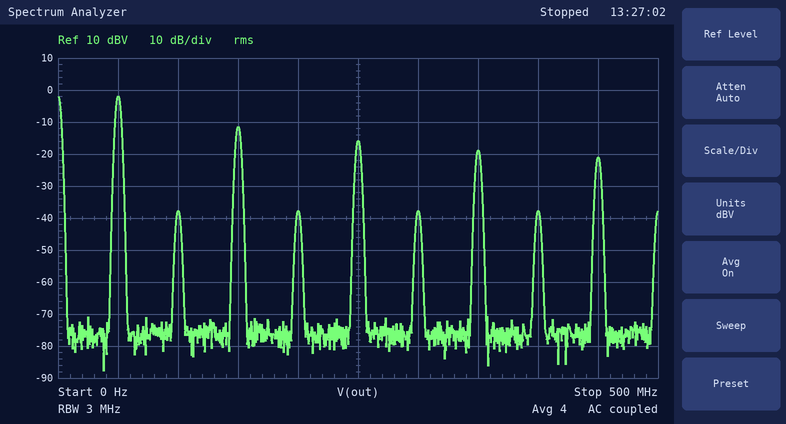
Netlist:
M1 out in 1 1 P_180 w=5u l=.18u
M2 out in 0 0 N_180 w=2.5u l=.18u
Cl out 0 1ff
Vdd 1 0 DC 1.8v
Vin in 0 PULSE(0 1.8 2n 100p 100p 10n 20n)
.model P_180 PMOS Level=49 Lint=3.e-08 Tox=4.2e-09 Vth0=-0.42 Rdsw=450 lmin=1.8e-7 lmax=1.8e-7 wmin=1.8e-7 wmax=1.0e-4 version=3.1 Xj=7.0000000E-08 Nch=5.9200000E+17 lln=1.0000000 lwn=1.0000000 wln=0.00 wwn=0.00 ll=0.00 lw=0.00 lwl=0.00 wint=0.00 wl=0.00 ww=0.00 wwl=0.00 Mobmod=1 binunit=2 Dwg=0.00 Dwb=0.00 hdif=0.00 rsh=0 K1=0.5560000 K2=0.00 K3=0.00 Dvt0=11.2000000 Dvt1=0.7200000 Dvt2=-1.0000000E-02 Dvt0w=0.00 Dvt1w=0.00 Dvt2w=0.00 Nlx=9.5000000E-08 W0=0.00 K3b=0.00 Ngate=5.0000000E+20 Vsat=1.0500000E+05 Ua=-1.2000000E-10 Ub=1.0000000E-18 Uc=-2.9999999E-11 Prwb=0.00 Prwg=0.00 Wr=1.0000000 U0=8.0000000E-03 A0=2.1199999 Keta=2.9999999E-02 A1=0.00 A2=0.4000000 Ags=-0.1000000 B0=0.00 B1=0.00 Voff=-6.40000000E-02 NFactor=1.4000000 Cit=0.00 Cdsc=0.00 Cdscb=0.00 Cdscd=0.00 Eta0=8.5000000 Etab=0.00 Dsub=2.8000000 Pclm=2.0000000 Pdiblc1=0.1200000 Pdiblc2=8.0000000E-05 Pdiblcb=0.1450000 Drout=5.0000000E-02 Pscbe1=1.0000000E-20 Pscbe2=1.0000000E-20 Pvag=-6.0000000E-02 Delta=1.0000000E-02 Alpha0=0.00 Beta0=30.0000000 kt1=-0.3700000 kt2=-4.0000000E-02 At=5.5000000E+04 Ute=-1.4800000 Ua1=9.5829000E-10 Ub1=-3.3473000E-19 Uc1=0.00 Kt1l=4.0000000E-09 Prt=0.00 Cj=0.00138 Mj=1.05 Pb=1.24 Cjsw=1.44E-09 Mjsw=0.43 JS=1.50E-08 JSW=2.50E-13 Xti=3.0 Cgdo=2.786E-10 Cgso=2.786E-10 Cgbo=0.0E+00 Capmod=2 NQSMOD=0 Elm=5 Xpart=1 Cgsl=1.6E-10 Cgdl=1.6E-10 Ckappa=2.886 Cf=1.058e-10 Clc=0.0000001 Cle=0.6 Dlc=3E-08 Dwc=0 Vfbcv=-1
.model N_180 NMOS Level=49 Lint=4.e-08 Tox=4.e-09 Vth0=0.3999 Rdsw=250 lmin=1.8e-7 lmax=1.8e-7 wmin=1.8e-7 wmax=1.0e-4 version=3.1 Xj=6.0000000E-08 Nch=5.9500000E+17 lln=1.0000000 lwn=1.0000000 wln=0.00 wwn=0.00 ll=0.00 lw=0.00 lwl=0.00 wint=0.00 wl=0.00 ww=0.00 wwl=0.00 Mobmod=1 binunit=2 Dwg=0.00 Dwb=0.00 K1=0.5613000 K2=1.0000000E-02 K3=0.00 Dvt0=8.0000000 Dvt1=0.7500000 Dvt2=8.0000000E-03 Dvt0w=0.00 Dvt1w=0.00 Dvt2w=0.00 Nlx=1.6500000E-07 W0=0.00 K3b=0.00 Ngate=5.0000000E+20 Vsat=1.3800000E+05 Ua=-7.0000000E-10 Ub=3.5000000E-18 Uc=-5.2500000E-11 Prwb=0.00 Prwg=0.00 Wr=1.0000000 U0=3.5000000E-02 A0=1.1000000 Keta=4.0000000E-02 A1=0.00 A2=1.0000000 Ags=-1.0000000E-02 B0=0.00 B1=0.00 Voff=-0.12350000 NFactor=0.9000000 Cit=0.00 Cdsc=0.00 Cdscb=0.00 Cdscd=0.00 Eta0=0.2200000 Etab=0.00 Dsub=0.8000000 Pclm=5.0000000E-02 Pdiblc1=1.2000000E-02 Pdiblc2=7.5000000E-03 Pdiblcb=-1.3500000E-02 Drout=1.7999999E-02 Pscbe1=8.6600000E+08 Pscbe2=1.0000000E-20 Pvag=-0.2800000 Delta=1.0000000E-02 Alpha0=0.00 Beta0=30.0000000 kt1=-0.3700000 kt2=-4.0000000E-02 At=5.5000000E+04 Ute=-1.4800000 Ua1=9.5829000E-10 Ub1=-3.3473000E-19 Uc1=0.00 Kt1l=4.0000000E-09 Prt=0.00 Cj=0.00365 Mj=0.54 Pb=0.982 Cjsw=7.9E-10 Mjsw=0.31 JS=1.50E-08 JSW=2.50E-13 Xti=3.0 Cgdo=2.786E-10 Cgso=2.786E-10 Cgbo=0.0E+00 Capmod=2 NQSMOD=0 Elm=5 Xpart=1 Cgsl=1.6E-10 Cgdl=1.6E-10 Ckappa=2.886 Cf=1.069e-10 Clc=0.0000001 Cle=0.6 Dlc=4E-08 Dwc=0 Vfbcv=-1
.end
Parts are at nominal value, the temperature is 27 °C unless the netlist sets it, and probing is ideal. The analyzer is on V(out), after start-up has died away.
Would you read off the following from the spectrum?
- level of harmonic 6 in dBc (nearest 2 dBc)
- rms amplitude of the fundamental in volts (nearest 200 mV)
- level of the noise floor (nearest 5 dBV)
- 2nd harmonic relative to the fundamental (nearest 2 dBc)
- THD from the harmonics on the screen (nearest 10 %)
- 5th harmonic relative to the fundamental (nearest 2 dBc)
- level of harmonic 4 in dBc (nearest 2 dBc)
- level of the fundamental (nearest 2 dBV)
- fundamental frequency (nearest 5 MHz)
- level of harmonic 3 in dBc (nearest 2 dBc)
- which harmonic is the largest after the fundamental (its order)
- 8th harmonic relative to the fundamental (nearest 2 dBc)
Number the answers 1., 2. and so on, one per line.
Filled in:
1. -36 dBc
2. 800 mV
3. -75 dBV
4. -36 dBc
5. 40 %
6. -14 dBc
7. -36 dBc
8. -2 dBV
9. 50 MHz
10. -10 dBc
11. 3
12. -36 dBc
